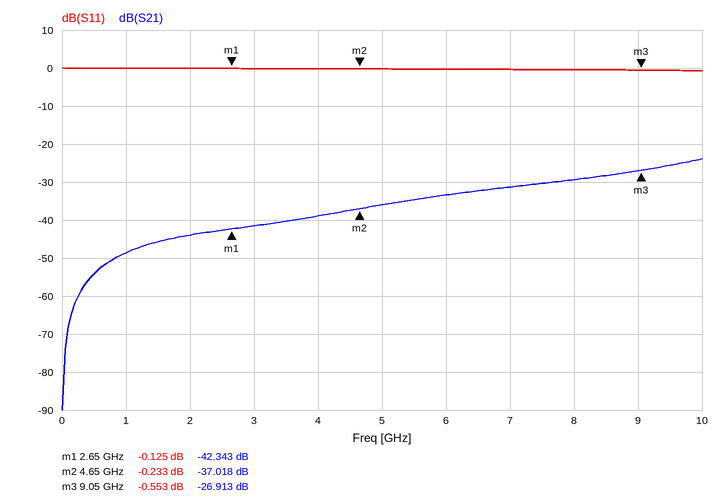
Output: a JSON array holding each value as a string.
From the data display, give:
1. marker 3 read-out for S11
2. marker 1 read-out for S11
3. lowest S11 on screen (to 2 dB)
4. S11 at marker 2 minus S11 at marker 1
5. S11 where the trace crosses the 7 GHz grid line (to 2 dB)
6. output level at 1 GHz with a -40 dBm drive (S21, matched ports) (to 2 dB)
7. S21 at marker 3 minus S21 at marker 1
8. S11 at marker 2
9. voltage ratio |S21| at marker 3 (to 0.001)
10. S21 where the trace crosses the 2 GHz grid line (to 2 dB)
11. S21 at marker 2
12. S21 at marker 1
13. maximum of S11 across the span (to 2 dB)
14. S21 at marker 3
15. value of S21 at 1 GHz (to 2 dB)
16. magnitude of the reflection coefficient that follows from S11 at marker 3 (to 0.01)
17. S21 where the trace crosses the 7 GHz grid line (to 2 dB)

["-0.553 dB", "-0.125 dB", "0 dB", "-0.108 dB", "0 dB", "-88 dBm", "15.430 dB", "-0.233 dB", "0.045", "-44 dB", "-37.018 dB", "-42.343 dB", "0 dB", "-26.913 dB", "-48 dB", "0.94", "-32 dB"]
